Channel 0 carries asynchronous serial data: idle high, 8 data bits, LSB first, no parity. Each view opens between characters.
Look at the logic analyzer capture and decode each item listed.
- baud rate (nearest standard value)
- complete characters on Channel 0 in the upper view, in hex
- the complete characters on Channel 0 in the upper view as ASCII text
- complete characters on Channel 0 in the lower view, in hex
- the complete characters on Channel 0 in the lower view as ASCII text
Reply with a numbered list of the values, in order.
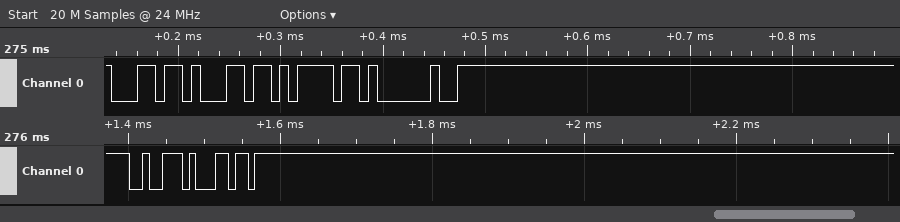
1. 115200 baud
2. 6C, 6C, 6F, 20
3. "llo "
4. 72, 6C
5. "rl"
